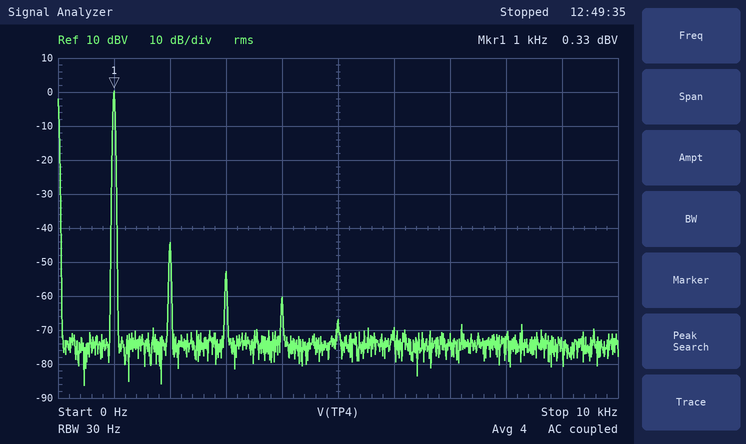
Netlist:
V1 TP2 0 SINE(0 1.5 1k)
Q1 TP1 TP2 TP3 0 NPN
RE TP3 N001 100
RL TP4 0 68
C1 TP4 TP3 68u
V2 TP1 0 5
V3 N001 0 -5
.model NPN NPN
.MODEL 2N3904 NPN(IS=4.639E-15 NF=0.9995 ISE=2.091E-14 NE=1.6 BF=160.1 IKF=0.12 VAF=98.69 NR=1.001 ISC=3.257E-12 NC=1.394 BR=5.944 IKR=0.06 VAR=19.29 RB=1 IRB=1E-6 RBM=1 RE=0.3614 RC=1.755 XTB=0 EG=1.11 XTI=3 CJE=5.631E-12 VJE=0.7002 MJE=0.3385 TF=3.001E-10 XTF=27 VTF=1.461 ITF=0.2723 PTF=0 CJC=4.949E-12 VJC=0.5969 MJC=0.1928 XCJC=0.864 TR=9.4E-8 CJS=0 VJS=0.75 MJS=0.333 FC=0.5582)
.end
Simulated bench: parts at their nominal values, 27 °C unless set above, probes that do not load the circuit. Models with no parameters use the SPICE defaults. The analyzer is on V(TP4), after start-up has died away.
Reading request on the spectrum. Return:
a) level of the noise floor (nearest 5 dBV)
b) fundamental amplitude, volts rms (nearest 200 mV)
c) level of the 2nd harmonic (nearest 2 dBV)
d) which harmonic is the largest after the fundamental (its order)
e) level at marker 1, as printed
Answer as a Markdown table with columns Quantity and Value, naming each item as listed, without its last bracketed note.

| Quantity | Value |
|---|---|
| level of the noise floor | -75 dBV |
| fundamental amplitude, volts rms | 1.0 V |
| level of the 2nd harmonic | -44 dBV |
| which harmonic is the largest after the fundamental | 2 |
| level at marker 1, as printed | 0.33 dBV |
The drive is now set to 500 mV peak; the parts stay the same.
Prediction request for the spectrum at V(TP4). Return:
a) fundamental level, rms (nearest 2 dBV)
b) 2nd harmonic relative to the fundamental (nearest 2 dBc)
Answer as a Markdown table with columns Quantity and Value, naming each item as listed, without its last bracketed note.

| Quantity | Value |
|---|---|
| fundamental level, rms | -10 dBV |
| 2nd harmonic relative to the fundamental | -58 dBc |
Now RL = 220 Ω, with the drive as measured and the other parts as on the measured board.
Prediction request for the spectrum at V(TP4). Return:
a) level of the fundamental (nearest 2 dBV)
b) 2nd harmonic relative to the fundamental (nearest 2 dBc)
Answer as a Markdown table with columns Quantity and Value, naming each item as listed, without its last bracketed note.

| Quantity | Value |
|---|---|
| level of the fundamental | 0 dBV |
| 2nd harmonic relative to the fundamental | -58 dBc |
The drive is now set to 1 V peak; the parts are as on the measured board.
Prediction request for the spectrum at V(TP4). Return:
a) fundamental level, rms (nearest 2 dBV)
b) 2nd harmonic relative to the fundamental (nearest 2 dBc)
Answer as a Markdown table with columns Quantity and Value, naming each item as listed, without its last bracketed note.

| Quantity | Value |
|---|---|
| fundamental level, rms | -4 dBV |
| 2nd harmonic relative to the fundamental | -52 dBc |
